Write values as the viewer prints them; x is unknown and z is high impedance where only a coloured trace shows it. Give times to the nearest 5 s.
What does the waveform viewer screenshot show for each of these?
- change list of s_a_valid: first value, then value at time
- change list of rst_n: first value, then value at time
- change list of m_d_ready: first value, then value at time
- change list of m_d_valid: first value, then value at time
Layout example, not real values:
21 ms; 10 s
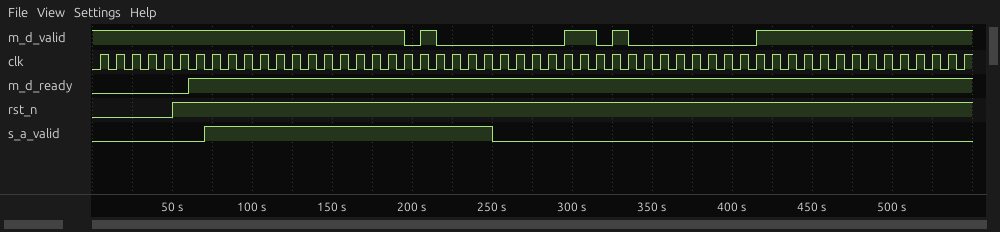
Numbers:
0, 1 at 70 s, 0 at 250 s; 0, 1 at 50 s; 0, 1 at 60 s; 1, 0 at 195 s, 1 at 205 s, 0 at 215 s, 1 at 295 s, 0 at 315 s, 1 at 325 s, 0 at 335 s, 1 at 415 s
